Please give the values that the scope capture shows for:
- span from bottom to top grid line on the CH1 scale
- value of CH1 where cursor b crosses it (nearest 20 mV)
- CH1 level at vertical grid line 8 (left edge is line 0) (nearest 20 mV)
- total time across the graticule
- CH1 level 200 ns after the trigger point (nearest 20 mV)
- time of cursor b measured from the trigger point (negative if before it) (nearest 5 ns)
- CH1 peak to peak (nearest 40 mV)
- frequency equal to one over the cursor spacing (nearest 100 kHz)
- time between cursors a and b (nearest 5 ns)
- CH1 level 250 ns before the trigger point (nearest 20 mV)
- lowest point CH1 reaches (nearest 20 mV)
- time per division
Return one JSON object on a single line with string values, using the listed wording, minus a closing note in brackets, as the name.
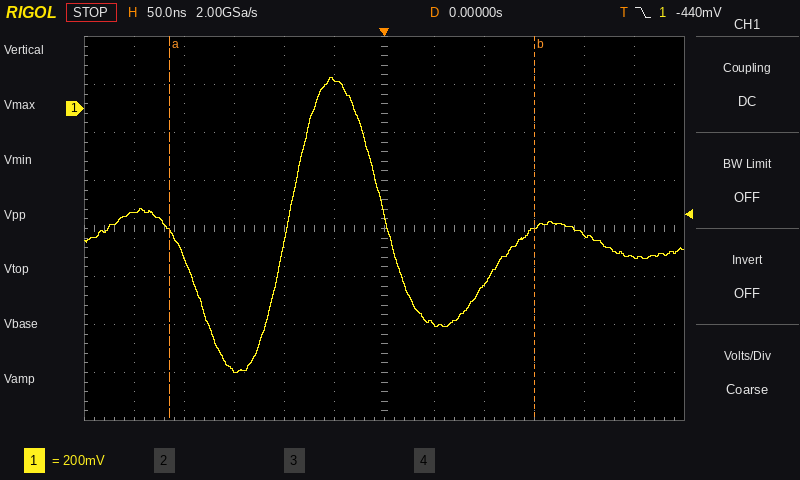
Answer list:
{"span from bottom to top grid line on the CH1 scale": "1.6 V", "value of CH1 where cursor b crosses it": "-500 mV", "CH1 level at vertical grid line 8 (left edge is line 0)": "-740 mV", "total time across the graticule": "600 ns", "CH1 level 200 ns after the trigger point": "-520 mV", "time of cursor b measured from the trigger point (negative if before it)": "+150 ns", "CH1 peak to peak": "1.24 V", "frequency equal to one over the cursor spacing": "2.7 MHz", "time between cursors a and b": "365 ns", "CH1 level 250 ns before the trigger point": "-440 mV", "lowest point CH1 reaches": "-1.10 V", "time per division": "50 ns"}
